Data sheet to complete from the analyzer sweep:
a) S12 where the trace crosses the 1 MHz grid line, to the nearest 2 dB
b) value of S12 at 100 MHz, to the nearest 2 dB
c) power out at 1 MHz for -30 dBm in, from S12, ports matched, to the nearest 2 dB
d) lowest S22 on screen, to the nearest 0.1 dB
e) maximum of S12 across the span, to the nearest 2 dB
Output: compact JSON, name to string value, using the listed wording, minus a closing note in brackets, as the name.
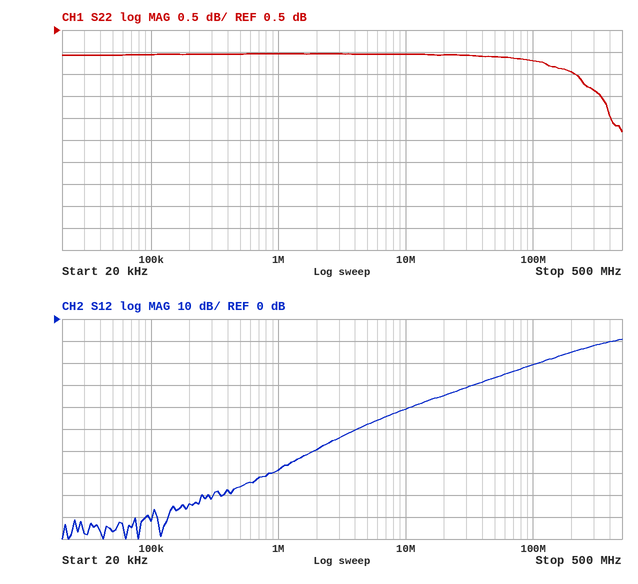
{"S12 where the trace crosses the 1 MHz grid line, to the nearest 2 dB": "-68 dB", "value of S12 at 100 MHz, to the nearest 2 dB": "-20 dB", "power out at 1 MHz for -30 dBm in, from S12, ports matched, to the nearest 2 dB": "-98 dBm", "lowest S22 on screen, to the nearest 0.1 dB": "-1.8 dB", "maximum of S12 across the span, to the nearest 2 dB": "-10 dB"}
